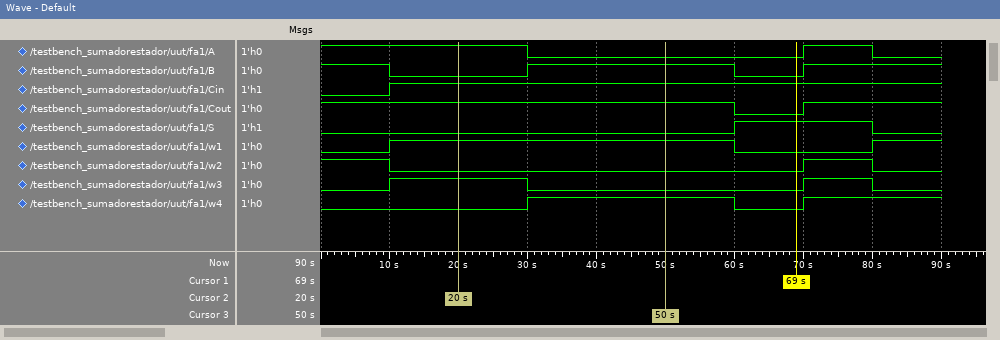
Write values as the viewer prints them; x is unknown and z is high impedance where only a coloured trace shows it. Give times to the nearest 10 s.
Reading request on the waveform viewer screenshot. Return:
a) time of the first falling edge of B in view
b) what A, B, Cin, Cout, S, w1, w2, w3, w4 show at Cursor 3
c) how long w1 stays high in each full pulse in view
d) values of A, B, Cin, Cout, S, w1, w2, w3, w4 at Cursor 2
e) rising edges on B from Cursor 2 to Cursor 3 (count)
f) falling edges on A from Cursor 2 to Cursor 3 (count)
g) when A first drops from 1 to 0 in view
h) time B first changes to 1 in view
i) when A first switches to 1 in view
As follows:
10 s
A=0, B=1, Cin=1, Cout=1, S=0, w1=1, w2=0, w3=0, w4=1
50 s
A=1, B=0, Cin=1, Cout=1, S=0, w1=1, w2=0, w3=1, w4=0
1
1
30 s
30 s
70 s
